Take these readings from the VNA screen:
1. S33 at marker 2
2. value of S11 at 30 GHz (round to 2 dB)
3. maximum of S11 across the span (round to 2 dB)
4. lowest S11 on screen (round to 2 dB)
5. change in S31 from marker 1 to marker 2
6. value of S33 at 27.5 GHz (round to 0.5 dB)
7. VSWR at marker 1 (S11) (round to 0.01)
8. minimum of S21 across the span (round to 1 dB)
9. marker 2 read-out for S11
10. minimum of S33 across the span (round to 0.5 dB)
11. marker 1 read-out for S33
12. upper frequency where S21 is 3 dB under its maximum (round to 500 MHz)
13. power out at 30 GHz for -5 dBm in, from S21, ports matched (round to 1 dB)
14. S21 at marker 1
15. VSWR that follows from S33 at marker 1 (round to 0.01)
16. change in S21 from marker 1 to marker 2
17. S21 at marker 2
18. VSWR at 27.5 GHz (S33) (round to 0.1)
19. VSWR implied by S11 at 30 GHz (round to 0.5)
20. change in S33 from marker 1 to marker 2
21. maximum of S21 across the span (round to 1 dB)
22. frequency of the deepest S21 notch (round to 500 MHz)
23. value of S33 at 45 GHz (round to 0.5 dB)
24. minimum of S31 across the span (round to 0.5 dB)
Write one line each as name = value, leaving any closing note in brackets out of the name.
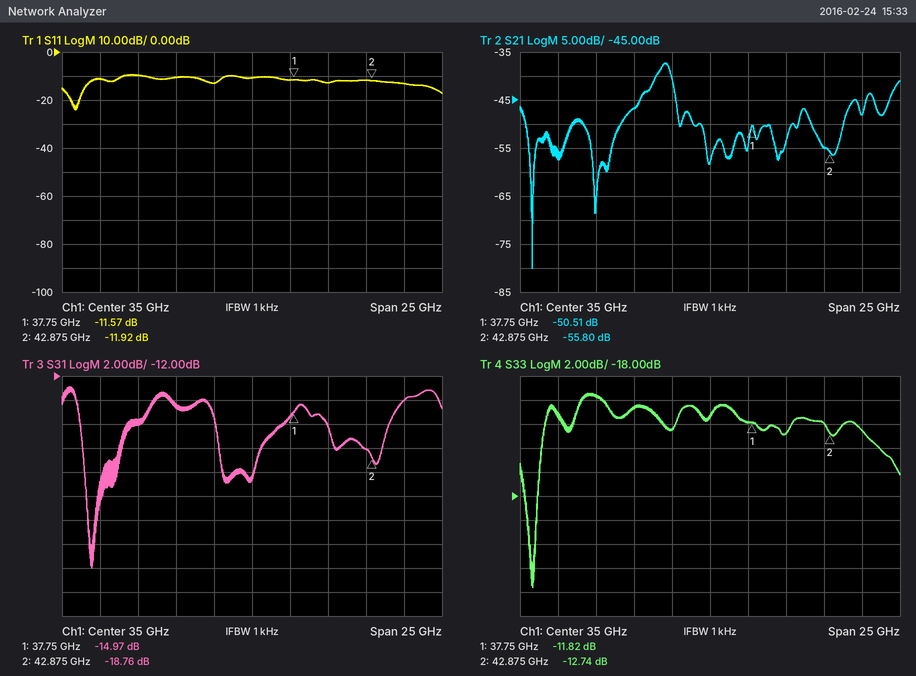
S33 at marker 2 = -12.74 dB
value of S11 at 30 GHz = -10 dB
maximum of S11 across the span = -10 dB
lowest S11 on screen = -24 dB
change in S31 from marker 1 to marker 2 = -3.79 dB
value of S33 at 27.5 GHz = -9.5 dB
VSWR at marker 1 (S11) = 1.72
minimum of S21 across the span = -80 dB
marker 2 read-out for S11 = -11.92 dB
minimum of S33 across the span = -25.5 dB
marker 1 read-out for S33 = -11.82 dB
upper frequency where S21 is 3 dB under its maximum = 32.5 GHz
power out at 30 GHz for -5 dBm in, from S21, ports matched = -52 dBm
S21 at marker 1 = -50.51 dB
VSWR that follows from S33 at marker 1 = 1.69
change in S21 from marker 1 to marker 2 = -5.29 dB
S21 at marker 2 = -55.80 dB
VSWR at 27.5 GHz (S33) = 2.0
VSWR implied by S11 at 30 GHz = 2.0
change in S33 from marker 1 to marker 2 = -0.92 dB
maximum of S21 across the span = -37 dB
frequency of the deepest S21 notch = 23.5 GHz
value of S33 at 45 GHz = -12.5 dB
minimum of S31 across the span = -28.0 dB
